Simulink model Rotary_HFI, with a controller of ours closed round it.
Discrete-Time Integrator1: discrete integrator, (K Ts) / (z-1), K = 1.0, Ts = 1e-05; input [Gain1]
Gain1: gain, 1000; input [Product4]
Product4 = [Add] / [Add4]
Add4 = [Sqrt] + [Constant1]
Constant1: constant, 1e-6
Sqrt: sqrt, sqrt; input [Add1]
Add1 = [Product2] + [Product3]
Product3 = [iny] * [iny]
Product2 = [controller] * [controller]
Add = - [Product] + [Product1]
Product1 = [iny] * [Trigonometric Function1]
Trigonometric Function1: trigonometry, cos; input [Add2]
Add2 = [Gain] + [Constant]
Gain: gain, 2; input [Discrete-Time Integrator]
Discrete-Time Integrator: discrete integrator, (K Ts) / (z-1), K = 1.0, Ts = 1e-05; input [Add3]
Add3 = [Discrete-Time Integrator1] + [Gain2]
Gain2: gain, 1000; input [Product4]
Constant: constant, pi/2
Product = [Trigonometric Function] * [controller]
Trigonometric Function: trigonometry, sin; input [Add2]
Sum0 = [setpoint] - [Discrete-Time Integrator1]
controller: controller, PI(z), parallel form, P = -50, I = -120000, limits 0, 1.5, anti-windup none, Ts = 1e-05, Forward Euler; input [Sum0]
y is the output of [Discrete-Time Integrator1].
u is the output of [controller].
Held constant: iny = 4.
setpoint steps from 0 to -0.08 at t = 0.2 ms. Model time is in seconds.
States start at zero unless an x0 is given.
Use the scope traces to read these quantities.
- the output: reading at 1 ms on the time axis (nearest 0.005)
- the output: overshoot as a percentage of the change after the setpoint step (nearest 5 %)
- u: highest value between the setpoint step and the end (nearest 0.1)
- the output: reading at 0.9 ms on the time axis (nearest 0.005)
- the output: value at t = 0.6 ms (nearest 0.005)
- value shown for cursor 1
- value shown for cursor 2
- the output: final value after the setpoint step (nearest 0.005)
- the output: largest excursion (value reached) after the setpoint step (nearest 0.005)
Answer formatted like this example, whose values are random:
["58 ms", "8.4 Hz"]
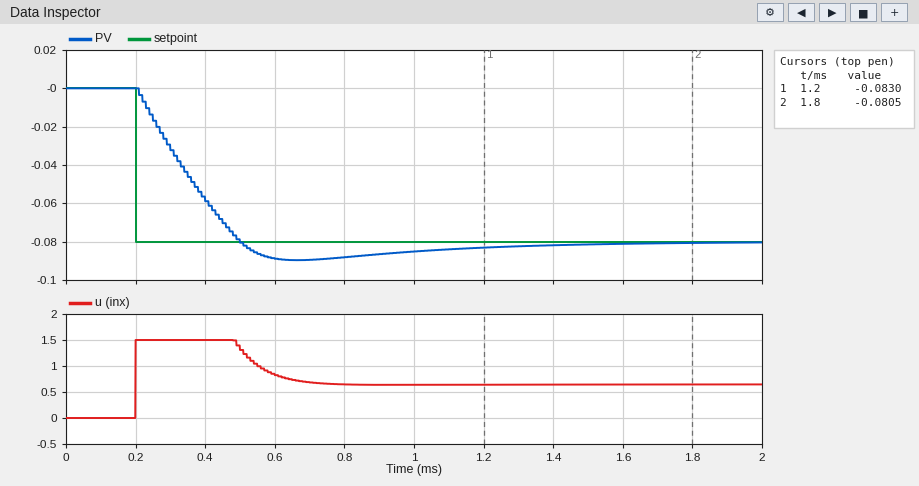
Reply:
["-0.085", "10 %", "1.5", "-0.085", "-0.090", "-0.0830", "-0.0805", "-0.080", "-0.090"]
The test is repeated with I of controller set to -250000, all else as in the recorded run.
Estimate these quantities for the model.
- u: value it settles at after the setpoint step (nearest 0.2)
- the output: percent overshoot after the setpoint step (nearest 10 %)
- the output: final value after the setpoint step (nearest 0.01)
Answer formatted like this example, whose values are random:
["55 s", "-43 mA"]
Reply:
["0.6", "30 %", "-0.08"]
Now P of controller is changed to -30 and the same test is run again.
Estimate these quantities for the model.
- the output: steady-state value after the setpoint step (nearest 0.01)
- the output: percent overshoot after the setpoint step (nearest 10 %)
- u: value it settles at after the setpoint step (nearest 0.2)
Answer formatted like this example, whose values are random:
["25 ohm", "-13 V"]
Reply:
["-0.08", "20 %", "0.6"]
